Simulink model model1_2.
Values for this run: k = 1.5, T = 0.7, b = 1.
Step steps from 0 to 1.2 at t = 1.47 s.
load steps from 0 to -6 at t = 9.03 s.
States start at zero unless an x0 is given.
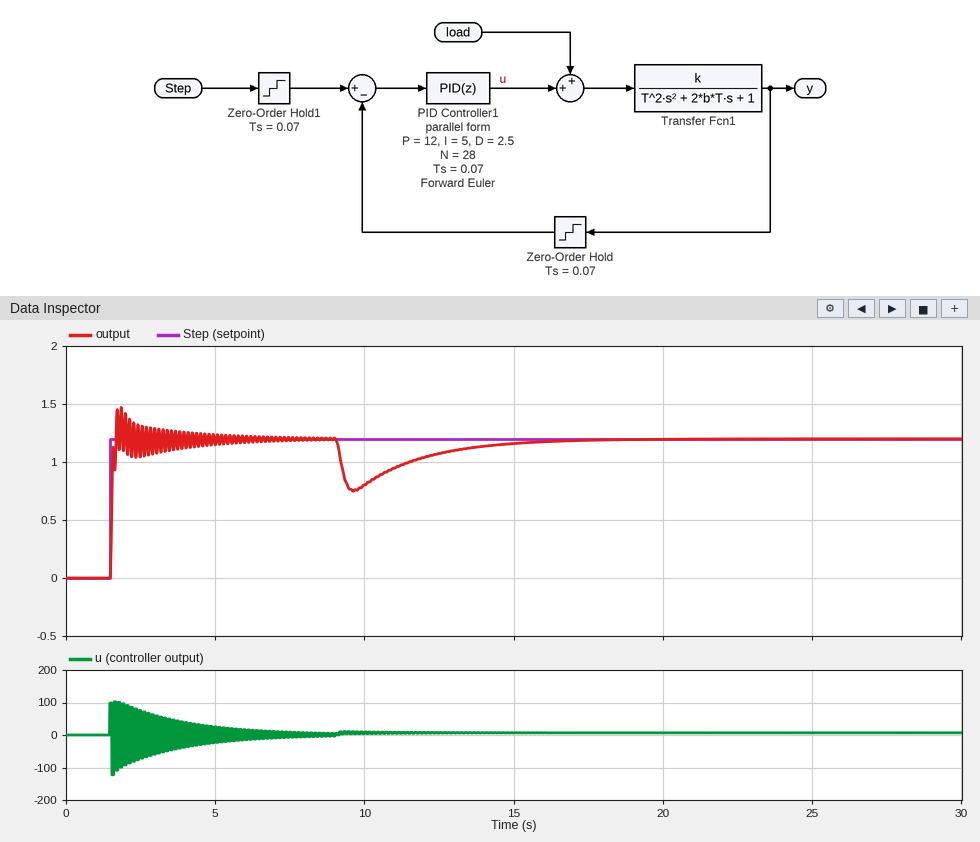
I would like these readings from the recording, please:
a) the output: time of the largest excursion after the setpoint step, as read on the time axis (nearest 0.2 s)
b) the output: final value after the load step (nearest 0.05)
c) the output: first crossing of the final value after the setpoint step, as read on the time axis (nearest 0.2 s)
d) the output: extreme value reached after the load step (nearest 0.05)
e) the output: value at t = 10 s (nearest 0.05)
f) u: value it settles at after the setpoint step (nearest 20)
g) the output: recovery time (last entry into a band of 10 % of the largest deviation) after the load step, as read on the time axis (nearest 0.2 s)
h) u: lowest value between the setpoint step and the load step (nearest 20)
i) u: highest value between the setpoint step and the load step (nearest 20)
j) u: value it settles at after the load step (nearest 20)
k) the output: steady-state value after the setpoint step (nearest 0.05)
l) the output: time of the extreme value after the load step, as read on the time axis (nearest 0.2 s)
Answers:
1.8 s
1.20
1.6 s
0.75
0.80
0
14.8 s
-120
100
0
1.20
9.6 s
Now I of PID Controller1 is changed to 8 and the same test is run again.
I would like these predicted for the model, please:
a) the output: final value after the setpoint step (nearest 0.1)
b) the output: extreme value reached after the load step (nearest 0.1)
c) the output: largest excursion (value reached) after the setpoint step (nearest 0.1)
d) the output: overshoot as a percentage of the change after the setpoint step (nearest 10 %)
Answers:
1.2
0.8
1.5
20 %
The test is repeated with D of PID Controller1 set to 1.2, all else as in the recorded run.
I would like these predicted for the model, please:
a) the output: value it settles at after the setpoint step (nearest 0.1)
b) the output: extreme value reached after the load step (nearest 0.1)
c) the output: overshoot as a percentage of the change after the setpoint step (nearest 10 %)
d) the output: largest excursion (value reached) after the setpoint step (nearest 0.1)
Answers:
1.2
0.6
30 %
1.6
